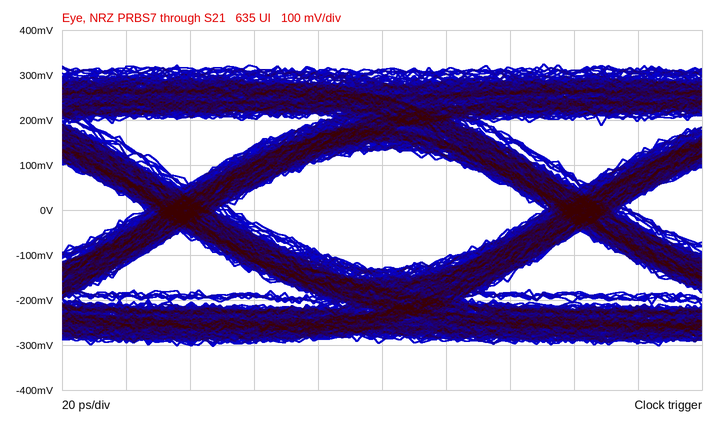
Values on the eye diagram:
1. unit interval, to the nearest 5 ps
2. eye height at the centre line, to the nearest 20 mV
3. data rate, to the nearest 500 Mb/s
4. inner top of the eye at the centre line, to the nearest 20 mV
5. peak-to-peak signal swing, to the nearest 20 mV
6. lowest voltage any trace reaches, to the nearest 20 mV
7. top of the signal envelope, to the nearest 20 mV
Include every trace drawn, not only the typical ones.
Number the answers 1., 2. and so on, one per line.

1. 125 ps
2. 260 mV
3. 8.0 Gb/s
4. 140 mV
5. 620 mV
6. -300 mV
7. 320 mV
